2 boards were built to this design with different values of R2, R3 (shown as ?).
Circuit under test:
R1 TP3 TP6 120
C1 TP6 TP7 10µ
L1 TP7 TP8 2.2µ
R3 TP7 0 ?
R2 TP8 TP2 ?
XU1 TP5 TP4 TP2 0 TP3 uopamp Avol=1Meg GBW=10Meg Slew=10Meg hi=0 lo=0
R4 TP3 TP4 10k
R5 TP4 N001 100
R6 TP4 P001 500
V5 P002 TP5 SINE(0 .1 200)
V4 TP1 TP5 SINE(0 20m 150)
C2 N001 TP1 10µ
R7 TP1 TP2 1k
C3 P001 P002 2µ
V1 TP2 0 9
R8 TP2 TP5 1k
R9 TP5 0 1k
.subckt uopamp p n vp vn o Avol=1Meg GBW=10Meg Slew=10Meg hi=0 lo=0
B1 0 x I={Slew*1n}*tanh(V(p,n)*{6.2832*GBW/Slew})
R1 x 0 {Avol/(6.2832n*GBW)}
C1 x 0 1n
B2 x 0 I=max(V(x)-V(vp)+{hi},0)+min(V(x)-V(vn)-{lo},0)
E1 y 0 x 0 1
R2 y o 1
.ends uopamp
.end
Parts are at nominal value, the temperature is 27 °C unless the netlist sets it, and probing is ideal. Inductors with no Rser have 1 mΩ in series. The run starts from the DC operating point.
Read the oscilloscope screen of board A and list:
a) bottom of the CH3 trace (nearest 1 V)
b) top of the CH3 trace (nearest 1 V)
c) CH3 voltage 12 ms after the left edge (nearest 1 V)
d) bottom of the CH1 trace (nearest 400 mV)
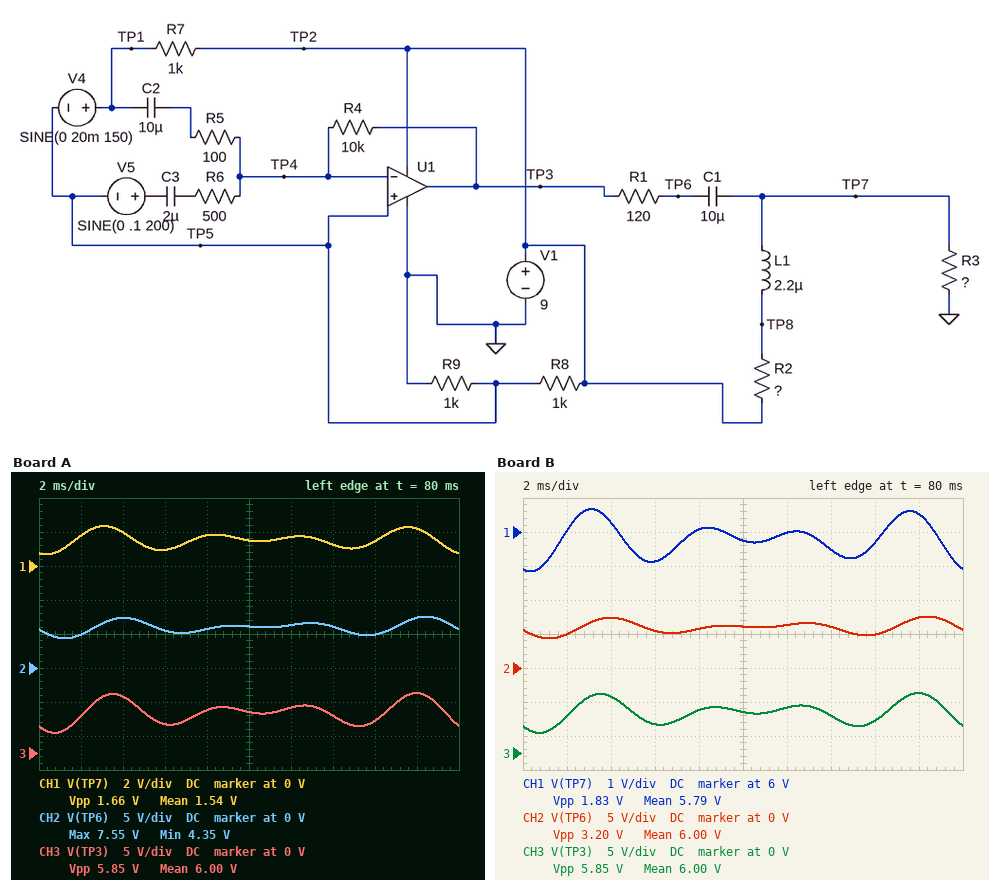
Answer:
3 V
9 V
7 V
800 mV
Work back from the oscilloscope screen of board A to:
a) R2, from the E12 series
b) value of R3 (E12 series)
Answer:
330 Ω
68 Ω
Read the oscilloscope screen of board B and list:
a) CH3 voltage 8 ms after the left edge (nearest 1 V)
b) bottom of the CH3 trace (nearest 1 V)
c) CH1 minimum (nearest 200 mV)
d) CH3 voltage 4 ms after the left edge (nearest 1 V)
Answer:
6 V
3 V
4.8 V
8 V
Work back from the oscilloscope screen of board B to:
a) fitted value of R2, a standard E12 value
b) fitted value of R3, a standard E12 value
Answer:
100 Ω
180 Ω
